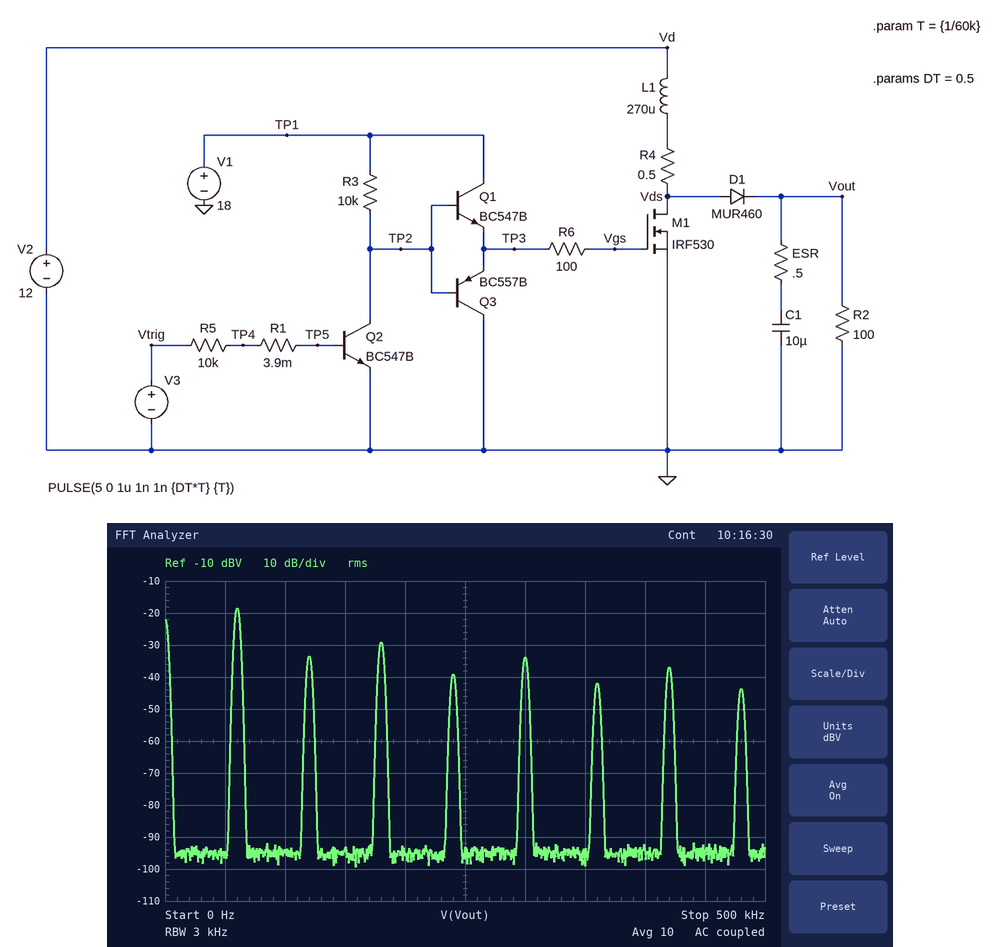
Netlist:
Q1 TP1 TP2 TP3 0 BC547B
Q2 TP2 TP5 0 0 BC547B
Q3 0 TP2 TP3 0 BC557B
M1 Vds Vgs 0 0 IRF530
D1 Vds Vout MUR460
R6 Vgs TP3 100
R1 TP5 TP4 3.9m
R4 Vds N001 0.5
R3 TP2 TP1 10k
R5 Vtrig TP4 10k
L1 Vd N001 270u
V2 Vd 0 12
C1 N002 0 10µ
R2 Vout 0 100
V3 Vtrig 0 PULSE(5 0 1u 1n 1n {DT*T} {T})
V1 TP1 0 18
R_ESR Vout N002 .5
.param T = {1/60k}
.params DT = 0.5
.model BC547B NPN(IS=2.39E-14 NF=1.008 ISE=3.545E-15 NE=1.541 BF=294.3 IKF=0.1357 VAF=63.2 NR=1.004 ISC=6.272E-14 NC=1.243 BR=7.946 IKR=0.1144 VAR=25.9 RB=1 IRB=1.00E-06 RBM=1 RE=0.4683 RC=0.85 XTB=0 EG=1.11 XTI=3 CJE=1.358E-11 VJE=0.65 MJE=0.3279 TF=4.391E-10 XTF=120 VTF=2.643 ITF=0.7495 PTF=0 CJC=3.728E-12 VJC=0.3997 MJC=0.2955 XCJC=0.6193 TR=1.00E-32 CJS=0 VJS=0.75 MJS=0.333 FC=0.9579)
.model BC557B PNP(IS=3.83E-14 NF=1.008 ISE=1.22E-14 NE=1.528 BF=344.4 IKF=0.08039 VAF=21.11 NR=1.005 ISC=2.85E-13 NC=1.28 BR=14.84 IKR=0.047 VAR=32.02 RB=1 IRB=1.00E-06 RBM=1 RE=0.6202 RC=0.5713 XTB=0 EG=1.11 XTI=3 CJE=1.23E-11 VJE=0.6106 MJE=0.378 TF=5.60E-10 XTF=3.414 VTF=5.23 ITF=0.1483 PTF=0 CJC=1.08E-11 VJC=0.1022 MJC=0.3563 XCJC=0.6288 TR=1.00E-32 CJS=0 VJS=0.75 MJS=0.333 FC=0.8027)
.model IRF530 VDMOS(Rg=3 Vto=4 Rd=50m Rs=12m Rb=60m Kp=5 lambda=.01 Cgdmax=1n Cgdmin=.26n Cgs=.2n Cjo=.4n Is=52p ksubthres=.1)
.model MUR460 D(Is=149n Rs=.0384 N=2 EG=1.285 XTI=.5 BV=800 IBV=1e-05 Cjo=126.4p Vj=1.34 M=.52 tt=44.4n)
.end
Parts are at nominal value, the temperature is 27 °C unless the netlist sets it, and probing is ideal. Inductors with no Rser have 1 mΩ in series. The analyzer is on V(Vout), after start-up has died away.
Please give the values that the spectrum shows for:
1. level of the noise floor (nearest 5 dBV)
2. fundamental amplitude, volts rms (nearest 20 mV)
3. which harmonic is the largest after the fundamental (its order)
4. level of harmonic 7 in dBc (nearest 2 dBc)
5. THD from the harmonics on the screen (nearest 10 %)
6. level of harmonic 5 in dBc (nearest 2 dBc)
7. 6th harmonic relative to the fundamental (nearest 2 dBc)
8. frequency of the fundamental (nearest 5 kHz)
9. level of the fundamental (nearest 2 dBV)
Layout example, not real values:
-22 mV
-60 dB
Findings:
-95 dBV
120 mV
3
-18 dBc
40 %
-16 dBc
-24 dBc
60 kHz
-18 dBV
